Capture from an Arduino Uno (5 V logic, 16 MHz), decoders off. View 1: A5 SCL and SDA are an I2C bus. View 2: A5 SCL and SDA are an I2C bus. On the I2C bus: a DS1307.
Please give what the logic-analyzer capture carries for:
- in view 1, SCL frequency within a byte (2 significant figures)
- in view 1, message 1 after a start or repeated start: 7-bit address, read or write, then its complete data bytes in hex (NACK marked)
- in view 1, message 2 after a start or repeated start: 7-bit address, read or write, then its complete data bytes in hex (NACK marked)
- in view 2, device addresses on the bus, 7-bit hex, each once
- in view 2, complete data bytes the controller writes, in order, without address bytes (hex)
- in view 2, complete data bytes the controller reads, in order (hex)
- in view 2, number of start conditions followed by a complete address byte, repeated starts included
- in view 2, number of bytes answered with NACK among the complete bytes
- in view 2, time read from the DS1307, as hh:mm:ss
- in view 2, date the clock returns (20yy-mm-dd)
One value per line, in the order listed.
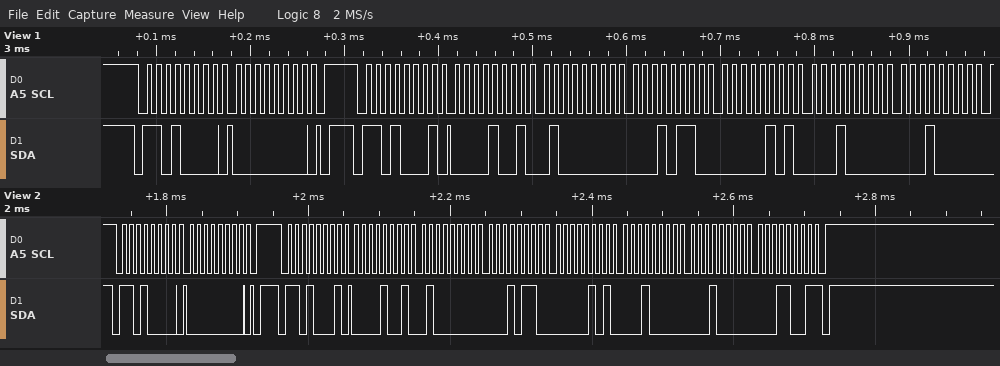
100 kHz
0x68 write: 00
0x68 read: 09 40 16 05 10 10
0x68
00
09 40 16 05 10 10 19
2
1
16:40:09
2019-10-10
